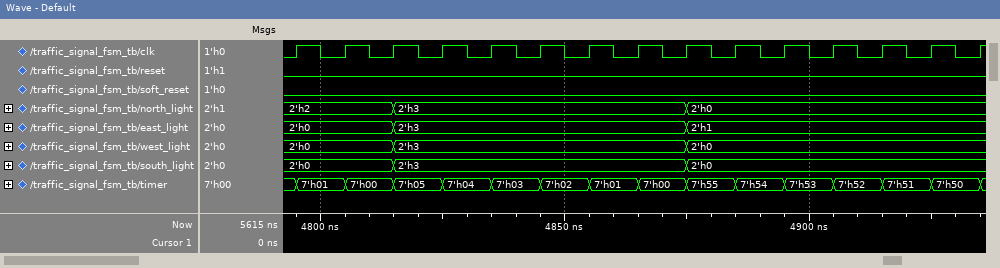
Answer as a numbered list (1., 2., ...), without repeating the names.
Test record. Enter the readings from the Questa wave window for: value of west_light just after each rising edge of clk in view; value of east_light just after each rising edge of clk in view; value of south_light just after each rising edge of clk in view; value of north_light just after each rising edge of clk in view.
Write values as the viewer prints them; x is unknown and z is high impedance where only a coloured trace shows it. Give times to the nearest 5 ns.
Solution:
1. 2'h0, 2'h0, 2'h3, 2'h3, 2'h3, 2'h3, 2'h3, 2'h3, 2'h0, 2'h0, 2'h0, 2'h0, 2'h0, 2'h0, 2'h0
2. 2'h0, 2'h0, 2'h3, 2'h3, 2'h3, 2'h3, 2'h3, 2'h3, 2'h1, 2'h1, 2'h1, 2'h1, 2'h1, 2'h1, 2'h1
3. 2'h0, 2'h0, 2'h3, 2'h3, 2'h3, 2'h3, 2'h3, 2'h3, 2'h0, 2'h0, 2'h0, 2'h0, 2'h0, 2'h0, 2'h0
4. 2'h2, 2'h2, 2'h3, 2'h3, 2'h3, 2'h3, 2'h3, 2'h3, 2'h0, 2'h0, 2'h0, 2'h0, 2'h0, 2'h0, 2'h0
